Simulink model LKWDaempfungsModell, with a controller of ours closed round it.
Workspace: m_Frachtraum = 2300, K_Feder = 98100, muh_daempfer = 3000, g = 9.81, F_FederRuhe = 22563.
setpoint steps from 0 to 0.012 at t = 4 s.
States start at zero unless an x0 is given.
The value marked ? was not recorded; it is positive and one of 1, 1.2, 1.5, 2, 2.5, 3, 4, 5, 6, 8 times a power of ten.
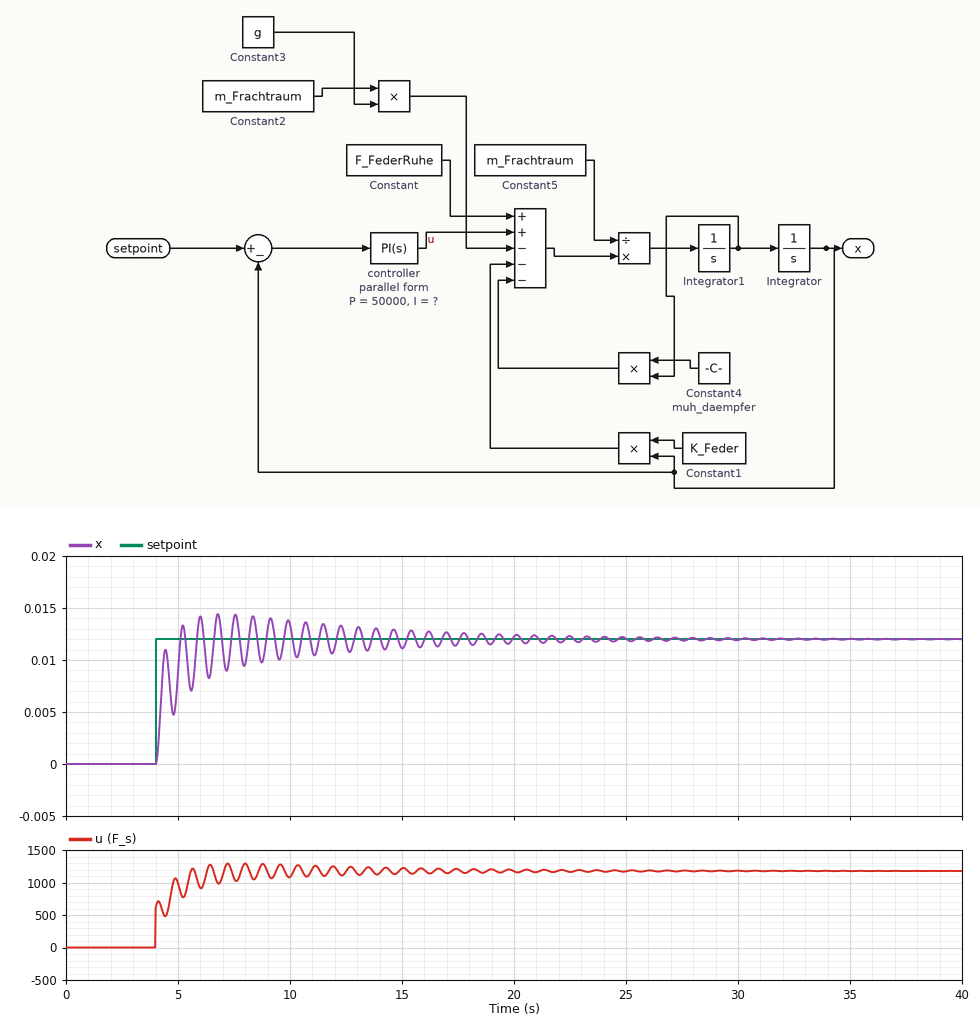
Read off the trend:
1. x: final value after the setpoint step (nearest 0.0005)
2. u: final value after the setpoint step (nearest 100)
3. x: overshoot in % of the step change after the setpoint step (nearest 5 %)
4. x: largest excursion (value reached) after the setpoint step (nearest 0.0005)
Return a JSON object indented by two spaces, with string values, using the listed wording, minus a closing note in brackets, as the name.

{
  "x: final value after the setpoint step": "0.0120",
  "u: final value after the setpoint step": "1200",
  "x: overshoot in % of the step change after the setpoint step": "20 %",
  "x: largest excursion (value reached) after the setpoint step": "0.0145"
}
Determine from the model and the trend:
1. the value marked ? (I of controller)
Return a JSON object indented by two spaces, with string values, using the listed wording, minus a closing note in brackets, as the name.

{
  "the value marked ?": "150000"
}
